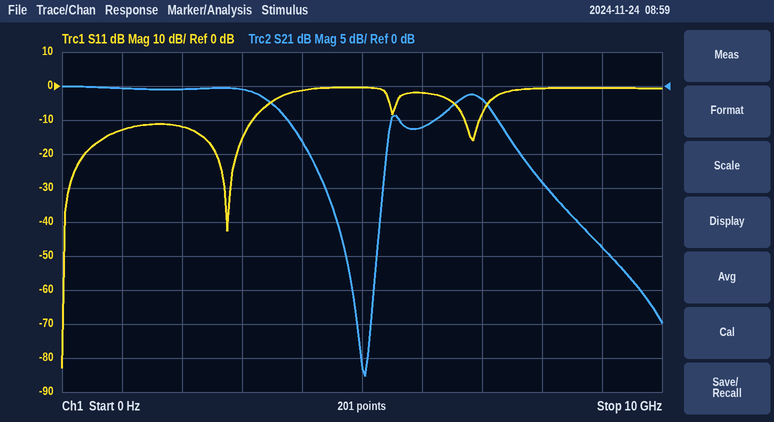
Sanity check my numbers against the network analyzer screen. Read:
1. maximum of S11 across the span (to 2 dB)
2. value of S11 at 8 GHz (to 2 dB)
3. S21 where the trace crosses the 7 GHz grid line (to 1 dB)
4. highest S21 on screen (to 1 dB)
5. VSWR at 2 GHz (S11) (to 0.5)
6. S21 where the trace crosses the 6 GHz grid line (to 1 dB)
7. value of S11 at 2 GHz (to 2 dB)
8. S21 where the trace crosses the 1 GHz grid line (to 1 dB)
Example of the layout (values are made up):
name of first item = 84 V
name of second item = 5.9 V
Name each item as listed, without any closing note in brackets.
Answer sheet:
maximum of S11 across the span = 0 dB
value of S11 at 8 GHz = 0 dB
S21 where the trace crosses the 7 GHz grid line = -2 dB
highest S21 on screen = 0 dB
VSWR at 2 GHz (S11) = 1.5
S21 where the trace crosses the 6 GHz grid line = -6 dB
value of S11 at 2 GHz = -12 dB
S21 where the trace crosses the 1 GHz grid line = 0 dB
